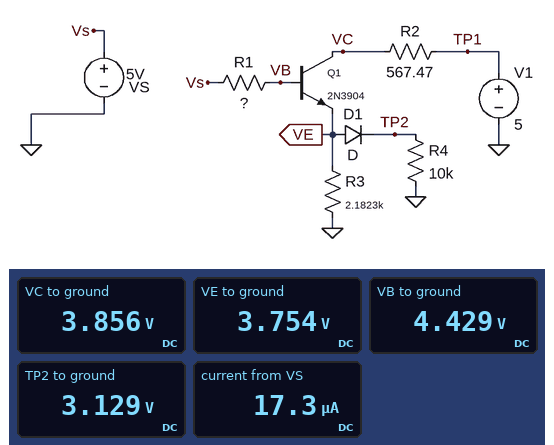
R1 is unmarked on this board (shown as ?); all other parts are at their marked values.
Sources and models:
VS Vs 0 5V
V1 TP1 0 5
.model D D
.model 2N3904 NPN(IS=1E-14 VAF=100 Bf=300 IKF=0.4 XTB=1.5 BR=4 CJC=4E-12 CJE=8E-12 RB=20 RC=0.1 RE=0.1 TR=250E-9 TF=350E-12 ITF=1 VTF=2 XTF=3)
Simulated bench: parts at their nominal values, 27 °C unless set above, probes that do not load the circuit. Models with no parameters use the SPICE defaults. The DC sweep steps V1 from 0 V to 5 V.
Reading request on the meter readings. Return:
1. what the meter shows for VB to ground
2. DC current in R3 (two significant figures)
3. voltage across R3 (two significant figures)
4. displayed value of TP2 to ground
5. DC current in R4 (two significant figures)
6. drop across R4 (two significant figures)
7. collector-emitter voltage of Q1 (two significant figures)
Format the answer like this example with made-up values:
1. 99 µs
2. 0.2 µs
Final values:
1. 4.429 V
2. 1.7 mA
3. 3.8 V
4. 3.129 V
5. 310 µA
6. 3.1 V
7. 100 mV
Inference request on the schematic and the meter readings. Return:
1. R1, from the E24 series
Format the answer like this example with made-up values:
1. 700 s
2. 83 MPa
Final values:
1. 33 kΩ
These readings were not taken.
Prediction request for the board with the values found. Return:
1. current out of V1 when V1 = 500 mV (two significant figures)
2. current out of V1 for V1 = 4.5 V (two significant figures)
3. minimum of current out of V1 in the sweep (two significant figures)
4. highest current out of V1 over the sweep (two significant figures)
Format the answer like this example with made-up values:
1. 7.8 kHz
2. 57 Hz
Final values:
1. 85 µA
2. 1.8 mA
3. -100 µA
4. 2.0 mA
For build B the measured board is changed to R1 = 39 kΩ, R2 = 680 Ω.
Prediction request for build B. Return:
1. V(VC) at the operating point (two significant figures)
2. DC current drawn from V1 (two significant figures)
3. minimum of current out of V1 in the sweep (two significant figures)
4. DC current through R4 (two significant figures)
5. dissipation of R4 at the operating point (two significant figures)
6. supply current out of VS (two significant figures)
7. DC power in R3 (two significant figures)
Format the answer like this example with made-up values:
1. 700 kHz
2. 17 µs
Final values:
1. 3.7 V
2. 1.9 mA
3. -85 µA
4. 300 µA
5. 880 µW
6. 19 µA
7. 5.9 mW
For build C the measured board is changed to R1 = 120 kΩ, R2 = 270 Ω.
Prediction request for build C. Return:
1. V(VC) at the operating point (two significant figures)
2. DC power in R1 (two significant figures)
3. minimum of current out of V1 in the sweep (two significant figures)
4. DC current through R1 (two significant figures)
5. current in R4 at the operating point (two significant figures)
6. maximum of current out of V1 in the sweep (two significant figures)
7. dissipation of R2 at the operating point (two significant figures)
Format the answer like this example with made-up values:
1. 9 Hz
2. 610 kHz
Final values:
1. 4.5 V
2. 4.9 µW
3. -33 µA
4. 6.4 µA
5. 290 µA
6. 1.9 mA
7. 990 µW
